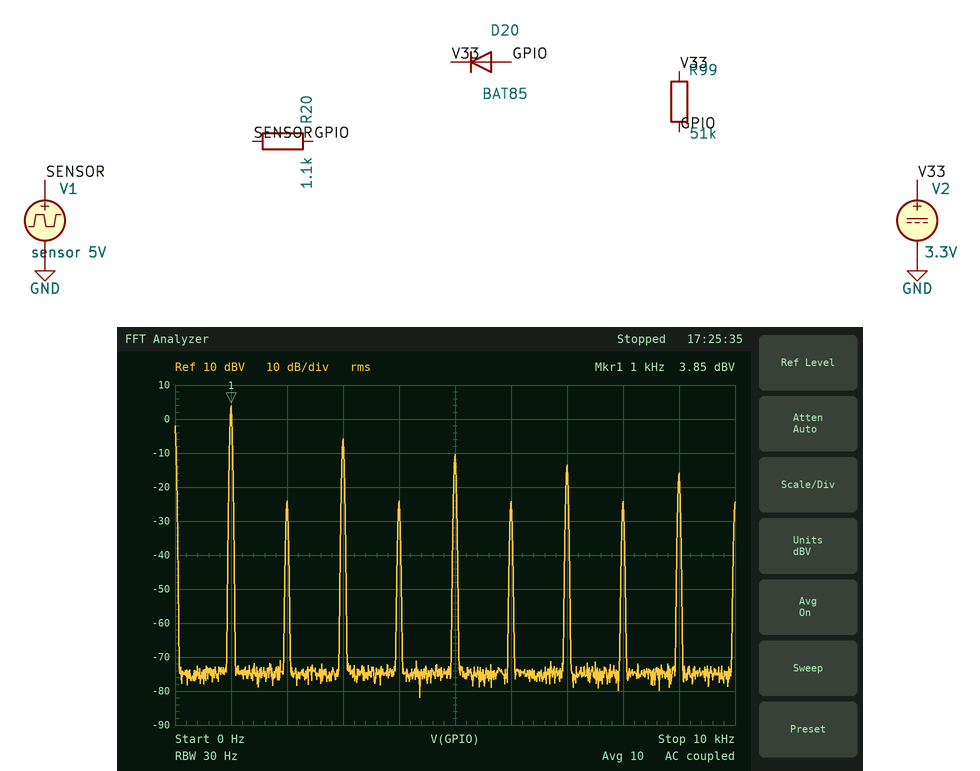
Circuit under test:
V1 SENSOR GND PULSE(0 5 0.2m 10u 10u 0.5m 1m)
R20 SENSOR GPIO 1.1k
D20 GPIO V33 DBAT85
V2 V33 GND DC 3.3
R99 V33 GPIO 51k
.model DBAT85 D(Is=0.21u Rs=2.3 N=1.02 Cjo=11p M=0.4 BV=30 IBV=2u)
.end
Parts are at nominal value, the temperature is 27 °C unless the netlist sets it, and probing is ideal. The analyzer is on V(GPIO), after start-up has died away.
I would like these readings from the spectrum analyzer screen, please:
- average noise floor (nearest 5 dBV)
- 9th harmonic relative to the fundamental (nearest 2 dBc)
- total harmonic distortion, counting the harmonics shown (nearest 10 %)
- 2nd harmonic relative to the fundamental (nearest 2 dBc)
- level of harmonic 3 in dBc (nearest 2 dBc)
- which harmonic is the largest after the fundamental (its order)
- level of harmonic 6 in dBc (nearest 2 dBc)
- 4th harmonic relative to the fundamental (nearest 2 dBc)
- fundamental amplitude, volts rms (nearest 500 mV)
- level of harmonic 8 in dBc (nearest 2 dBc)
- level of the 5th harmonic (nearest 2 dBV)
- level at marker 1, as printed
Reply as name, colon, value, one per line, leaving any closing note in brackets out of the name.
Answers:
average noise floor: -75 dBV
9th harmonic relative to the fundamental: -20 dBc
total harmonic distortion, counting the harmonics shown: 40 %
2nd harmonic relative to the fundamental: -28 dBc
level of harmonic 3 in dBc: -10 dBc
which harmonic is the largest after the fundamental: 3
level of harmonic 6 in dBc: -28 dBc
4th harmonic relative to the fundamental: -28 dBc
fundamental amplitude, volts rms: 1.5 V
level of harmonic 8 in dBc: -28 dBc
level of the 5th harmonic: -10 dBV
level at marker 1, as printed: 3.85 dBV
